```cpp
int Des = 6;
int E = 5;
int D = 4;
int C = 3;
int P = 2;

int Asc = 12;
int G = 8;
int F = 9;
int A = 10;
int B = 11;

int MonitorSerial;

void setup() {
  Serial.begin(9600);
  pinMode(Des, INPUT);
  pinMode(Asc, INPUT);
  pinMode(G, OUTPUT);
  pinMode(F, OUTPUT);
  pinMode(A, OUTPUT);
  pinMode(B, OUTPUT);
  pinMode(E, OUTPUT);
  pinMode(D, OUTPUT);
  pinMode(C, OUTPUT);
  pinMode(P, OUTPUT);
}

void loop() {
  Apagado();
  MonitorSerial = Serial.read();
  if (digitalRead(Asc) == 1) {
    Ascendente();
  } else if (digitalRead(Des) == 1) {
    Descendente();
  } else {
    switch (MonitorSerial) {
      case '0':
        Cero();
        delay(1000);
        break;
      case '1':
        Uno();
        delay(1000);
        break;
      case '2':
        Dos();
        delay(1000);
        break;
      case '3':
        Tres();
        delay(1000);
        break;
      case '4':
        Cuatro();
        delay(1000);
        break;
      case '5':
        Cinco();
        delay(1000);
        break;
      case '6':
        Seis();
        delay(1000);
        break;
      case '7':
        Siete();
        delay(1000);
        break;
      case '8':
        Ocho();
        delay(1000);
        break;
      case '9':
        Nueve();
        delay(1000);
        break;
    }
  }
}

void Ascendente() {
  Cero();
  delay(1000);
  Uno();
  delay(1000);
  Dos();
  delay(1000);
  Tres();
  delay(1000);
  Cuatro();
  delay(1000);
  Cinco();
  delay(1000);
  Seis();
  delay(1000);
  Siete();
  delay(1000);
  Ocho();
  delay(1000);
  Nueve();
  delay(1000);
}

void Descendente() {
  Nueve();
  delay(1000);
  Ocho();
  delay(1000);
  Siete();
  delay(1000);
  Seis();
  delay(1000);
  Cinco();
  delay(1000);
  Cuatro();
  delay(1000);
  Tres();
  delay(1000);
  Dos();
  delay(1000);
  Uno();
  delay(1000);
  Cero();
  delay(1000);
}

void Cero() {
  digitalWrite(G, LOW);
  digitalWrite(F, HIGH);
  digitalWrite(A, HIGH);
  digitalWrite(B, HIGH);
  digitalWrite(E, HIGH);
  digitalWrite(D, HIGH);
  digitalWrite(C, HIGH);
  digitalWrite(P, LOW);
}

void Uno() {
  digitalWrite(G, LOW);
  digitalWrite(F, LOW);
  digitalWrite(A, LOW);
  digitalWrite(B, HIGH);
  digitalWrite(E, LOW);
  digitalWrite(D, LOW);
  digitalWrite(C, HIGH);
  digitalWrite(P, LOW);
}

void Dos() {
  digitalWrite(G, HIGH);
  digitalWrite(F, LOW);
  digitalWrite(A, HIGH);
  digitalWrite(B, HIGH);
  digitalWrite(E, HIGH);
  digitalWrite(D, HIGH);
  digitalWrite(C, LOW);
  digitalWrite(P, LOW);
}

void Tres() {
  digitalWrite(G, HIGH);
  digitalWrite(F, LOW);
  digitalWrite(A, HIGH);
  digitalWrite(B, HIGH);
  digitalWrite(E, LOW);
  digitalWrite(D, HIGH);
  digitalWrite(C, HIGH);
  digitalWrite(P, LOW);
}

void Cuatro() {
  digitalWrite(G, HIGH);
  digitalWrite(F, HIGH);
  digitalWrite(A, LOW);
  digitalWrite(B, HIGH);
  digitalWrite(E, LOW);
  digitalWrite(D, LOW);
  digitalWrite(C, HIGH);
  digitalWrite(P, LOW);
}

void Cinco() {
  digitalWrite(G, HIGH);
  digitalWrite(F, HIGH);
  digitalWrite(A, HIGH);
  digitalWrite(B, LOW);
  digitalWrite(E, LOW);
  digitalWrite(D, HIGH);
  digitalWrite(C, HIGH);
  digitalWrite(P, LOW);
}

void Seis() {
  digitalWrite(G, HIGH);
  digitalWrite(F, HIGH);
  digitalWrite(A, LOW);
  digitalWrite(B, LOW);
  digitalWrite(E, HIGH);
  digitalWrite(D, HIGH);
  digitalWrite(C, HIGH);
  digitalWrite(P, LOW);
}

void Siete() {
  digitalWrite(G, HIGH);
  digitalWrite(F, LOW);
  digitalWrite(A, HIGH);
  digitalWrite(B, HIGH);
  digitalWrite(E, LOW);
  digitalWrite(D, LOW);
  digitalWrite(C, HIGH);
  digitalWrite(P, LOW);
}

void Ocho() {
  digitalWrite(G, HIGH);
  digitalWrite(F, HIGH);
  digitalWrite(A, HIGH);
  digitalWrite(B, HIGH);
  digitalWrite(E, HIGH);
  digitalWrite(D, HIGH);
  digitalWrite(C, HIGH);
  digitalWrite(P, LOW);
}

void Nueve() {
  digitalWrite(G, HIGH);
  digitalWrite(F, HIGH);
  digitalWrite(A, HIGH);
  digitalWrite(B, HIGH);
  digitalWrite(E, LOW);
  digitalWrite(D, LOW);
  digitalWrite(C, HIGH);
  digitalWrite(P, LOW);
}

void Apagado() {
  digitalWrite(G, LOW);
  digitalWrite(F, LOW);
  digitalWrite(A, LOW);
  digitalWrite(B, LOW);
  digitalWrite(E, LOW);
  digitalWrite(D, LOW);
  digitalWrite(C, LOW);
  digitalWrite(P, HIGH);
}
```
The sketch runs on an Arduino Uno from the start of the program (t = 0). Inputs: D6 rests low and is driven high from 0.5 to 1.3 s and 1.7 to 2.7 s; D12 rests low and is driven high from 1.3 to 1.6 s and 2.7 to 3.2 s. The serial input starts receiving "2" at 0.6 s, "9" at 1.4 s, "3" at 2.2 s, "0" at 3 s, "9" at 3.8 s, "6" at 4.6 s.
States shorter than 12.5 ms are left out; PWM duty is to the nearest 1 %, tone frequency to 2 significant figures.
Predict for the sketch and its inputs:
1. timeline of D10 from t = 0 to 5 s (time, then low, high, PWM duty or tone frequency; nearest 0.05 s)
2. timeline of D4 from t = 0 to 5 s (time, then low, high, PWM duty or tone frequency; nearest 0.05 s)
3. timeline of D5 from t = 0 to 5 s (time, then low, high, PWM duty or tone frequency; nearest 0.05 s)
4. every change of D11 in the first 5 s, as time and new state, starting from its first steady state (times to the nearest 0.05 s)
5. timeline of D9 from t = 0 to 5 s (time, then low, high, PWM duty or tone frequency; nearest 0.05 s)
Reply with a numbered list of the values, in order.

1. 0 s low; 0.5 s high; 3.5 s low; 4.5 s high
2. 0 s low; 1.5 s high; 2.5 s low; 3.5 s high
3. 0 s low; 1.5 s high; 2.5 s low; 3.5 s high; 4.5 s low
4. 0 s low; 0.5 s high; 3.5 s low
5. 0 s low; 0.5 s high; 2.5 s low; 3.5 s high
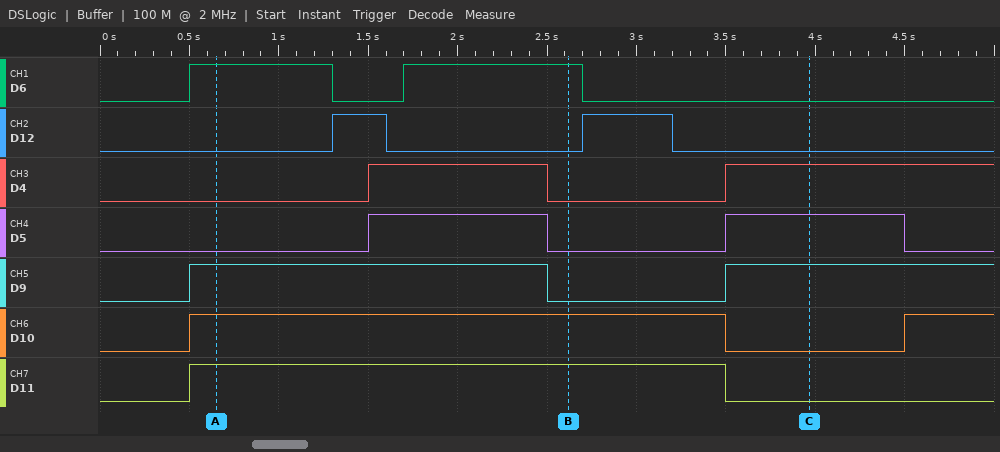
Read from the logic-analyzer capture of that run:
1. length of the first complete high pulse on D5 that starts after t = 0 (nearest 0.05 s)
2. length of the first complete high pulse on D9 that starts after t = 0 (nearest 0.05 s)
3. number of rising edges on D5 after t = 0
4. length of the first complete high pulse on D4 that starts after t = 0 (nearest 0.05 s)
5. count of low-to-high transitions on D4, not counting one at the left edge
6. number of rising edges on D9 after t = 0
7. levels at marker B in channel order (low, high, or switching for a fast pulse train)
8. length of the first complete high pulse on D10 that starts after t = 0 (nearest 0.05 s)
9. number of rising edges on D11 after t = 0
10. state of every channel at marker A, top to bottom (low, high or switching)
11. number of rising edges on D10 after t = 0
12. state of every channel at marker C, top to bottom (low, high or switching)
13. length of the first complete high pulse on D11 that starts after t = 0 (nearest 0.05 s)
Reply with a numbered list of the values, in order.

1. 1.00 s
2. 2.00 s
3. 2
4. 1.00 s
5. 2
6. 2
7. D6 high, D12 low, D4 low, D5 low, D9 low, D10 high, D11 high
8. 3.00 s
9. 1
10. D6 high, D12 low, D4 low, D5 low, D9 high, D10 high, D11 high
11. 2
12. D6 low, D12 low, D4 high, D5 high, D9 high, D10 low, D11 low
13. 3.00 s
